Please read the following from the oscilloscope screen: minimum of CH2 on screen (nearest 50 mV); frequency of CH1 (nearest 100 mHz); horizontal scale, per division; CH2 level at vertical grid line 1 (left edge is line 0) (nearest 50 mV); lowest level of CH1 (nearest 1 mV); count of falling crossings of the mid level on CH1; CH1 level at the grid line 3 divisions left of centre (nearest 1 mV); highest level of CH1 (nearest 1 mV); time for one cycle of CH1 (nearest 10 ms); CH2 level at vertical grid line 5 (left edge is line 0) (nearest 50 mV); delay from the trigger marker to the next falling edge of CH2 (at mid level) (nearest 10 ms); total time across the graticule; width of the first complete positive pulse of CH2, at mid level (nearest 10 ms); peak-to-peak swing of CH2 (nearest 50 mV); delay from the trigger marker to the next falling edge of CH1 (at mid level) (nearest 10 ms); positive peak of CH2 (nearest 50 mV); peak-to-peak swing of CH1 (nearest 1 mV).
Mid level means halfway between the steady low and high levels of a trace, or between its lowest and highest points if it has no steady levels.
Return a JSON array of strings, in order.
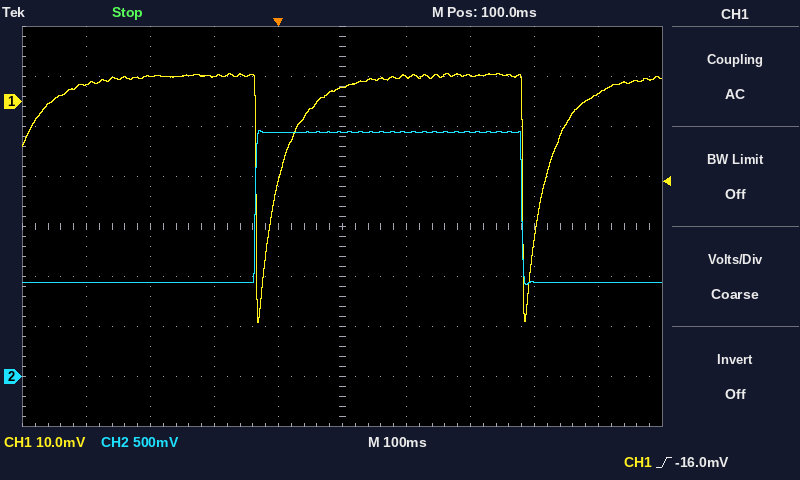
["900 mV", "2.4 Hz", "100 ms", "950 mV", "-44 mV", "2", "5 mV", "6 mV", "420 ms", "2.45 V", "380 ms", "1 s", "420 ms", "1.55 V", "380 ms", "2.45 V", "50 mV"]
